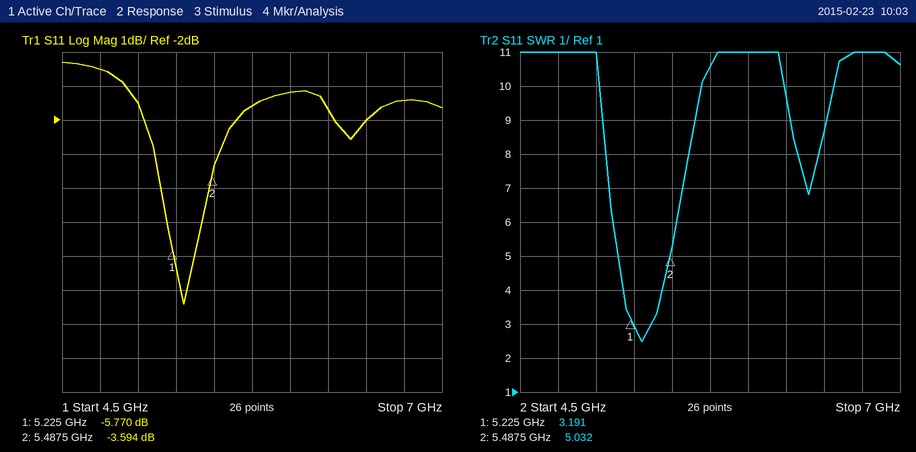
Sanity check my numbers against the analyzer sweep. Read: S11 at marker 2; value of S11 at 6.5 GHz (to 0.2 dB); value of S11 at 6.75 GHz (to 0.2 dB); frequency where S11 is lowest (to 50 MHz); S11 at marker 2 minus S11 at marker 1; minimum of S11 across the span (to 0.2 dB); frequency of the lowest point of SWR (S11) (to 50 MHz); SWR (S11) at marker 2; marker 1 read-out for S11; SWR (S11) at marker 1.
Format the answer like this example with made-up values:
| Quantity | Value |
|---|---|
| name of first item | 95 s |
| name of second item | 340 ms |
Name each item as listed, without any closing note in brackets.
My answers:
| Quantity | Value |
|---|---|
| S11 at marker 2 | -3.594 dB |
| value of S11 at 6.5 GHz | -2.0 dB |
| value of S11 at 6.75 GHz | -1.4 dB |
| frequency where S11 is lowest | 5.30 GHz |
| S11 at marker 2 minus S11 at marker 1 | 2.176 dB |
| minimum of S11 across the span | -7.4 dB |
| frequency of the lowest point of SWR (S11) | 5.30 GHz |
| SWR (S11) at marker 2 | 5.032 |
| marker 1 read-out for S11 | -5.770 dB |
| SWR (S11) at marker 1 | 3.191 |
